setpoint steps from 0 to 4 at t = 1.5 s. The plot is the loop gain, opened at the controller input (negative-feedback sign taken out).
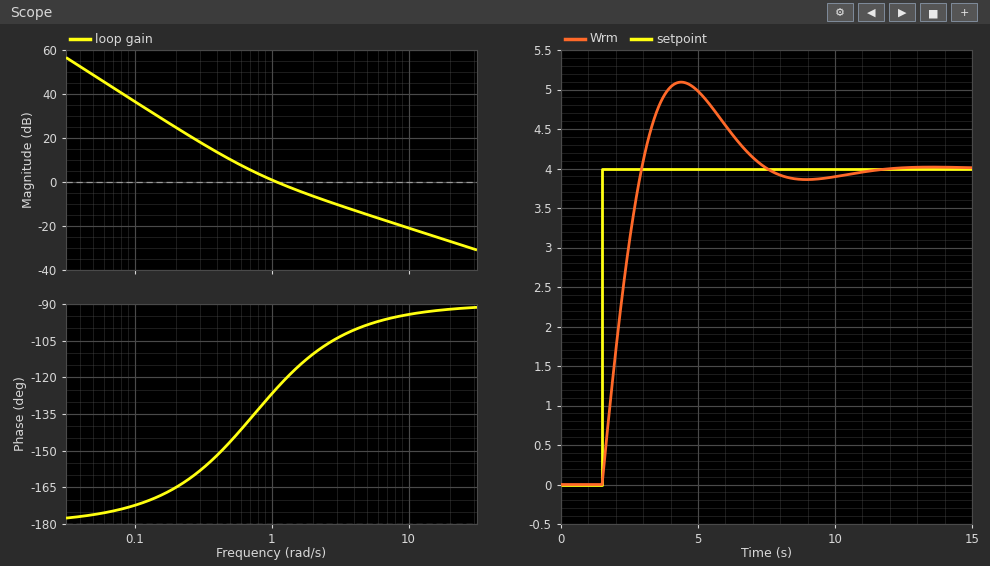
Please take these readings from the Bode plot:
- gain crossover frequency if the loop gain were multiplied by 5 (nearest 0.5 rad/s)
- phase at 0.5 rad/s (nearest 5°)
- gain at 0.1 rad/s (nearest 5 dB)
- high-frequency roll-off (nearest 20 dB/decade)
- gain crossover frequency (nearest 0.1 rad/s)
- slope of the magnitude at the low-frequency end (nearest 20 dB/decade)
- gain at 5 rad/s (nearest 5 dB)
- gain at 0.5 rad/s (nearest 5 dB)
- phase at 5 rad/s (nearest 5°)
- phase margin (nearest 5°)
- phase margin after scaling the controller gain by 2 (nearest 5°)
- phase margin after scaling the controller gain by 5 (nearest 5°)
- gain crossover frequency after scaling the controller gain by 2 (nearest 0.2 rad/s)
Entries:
4.5 rad/s
-145°
35 dB
-20 dB/decade
1.1 rad/s
-40 dB/decade
-15 dB
10 dB
-100°
55°
70°
80°
2.0 rad/s
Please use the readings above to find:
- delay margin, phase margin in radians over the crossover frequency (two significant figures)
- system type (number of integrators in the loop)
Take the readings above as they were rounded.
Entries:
0.87 s
2
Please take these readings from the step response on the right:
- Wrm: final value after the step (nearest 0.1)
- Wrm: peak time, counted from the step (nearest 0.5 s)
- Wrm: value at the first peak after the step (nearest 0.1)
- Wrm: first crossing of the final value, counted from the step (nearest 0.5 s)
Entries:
4.0
3.0 s
5.1
1.5 s
